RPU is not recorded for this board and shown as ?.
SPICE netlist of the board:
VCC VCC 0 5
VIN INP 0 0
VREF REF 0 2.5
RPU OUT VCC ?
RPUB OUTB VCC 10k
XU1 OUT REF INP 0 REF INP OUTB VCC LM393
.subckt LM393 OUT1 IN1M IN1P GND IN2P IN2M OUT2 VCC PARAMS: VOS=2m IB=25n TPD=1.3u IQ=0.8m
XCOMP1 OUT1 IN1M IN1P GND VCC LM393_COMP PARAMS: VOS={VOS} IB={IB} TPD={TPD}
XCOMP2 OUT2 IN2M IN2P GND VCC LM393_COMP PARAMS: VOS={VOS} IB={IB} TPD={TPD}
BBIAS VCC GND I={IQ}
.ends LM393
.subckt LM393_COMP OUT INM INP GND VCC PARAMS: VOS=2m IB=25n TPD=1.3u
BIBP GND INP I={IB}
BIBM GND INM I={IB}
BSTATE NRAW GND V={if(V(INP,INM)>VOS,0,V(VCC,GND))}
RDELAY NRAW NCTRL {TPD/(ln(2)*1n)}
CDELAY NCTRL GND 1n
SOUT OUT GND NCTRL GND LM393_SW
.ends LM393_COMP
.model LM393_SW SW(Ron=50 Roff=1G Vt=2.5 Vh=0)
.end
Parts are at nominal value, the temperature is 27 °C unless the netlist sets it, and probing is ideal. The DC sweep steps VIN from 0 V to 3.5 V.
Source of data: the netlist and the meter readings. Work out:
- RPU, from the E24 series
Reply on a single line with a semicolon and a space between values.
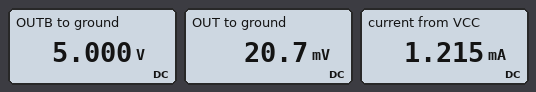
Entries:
12 kΩ
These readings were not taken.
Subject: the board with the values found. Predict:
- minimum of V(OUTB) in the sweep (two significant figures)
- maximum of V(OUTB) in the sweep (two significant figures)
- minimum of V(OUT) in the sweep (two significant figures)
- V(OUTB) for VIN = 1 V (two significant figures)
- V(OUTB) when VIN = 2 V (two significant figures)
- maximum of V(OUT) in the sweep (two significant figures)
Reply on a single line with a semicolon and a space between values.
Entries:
25 mV; 5.0 V; 21 mV; 5.0 V; 5.0 V; 5.0 V
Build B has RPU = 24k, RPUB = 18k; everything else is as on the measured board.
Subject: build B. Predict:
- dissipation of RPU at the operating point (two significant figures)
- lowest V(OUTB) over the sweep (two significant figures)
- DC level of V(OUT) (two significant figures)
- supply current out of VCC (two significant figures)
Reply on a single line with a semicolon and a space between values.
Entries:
1.0 mW; 14 mV; 10 mV; 1.0 mA
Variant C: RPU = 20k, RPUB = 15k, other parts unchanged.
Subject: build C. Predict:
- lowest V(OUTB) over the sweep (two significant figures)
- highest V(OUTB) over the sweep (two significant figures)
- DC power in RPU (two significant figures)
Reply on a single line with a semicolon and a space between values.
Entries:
17 mV; 5.0 V; 1.2 mW
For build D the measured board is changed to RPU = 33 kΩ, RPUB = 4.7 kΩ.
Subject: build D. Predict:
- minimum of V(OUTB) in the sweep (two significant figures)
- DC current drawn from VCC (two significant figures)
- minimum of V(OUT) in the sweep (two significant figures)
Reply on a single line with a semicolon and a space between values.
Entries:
53 mV; 950 µA; 7.6 mV
